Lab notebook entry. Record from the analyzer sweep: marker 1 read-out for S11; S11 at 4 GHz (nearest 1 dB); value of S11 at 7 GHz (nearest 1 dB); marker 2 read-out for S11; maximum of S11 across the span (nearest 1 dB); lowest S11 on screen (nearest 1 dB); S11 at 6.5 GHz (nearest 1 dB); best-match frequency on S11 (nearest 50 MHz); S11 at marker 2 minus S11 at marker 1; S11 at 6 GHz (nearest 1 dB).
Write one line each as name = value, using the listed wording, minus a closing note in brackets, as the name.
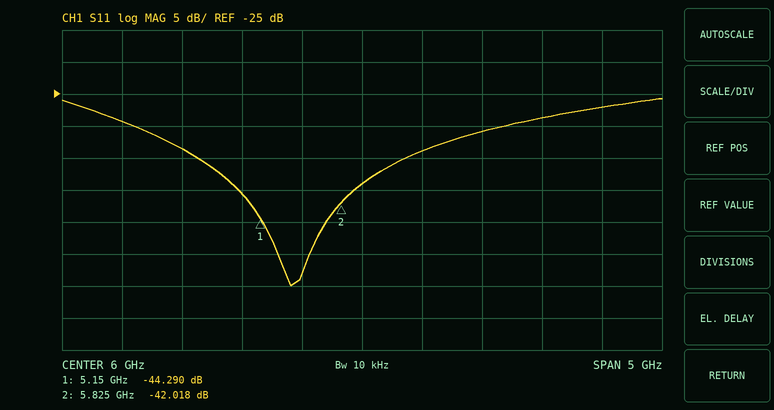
marker 1 read-out for S11 = -44.290 dB
S11 at 4 GHz = -29 dB
value of S11 at 7 GHz = -31 dB
marker 2 read-out for S11 = -42.018 dB
maximum of S11 across the span = -26 dB
lowest S11 on screen = -55 dB
S11 at 6.5 GHz = -34 dB
best-match frequency on S11 = 5.40 GHz
S11 at marker 2 minus S11 at marker 1 = 2.272 dB
S11 at 6 GHz = -39 dB
